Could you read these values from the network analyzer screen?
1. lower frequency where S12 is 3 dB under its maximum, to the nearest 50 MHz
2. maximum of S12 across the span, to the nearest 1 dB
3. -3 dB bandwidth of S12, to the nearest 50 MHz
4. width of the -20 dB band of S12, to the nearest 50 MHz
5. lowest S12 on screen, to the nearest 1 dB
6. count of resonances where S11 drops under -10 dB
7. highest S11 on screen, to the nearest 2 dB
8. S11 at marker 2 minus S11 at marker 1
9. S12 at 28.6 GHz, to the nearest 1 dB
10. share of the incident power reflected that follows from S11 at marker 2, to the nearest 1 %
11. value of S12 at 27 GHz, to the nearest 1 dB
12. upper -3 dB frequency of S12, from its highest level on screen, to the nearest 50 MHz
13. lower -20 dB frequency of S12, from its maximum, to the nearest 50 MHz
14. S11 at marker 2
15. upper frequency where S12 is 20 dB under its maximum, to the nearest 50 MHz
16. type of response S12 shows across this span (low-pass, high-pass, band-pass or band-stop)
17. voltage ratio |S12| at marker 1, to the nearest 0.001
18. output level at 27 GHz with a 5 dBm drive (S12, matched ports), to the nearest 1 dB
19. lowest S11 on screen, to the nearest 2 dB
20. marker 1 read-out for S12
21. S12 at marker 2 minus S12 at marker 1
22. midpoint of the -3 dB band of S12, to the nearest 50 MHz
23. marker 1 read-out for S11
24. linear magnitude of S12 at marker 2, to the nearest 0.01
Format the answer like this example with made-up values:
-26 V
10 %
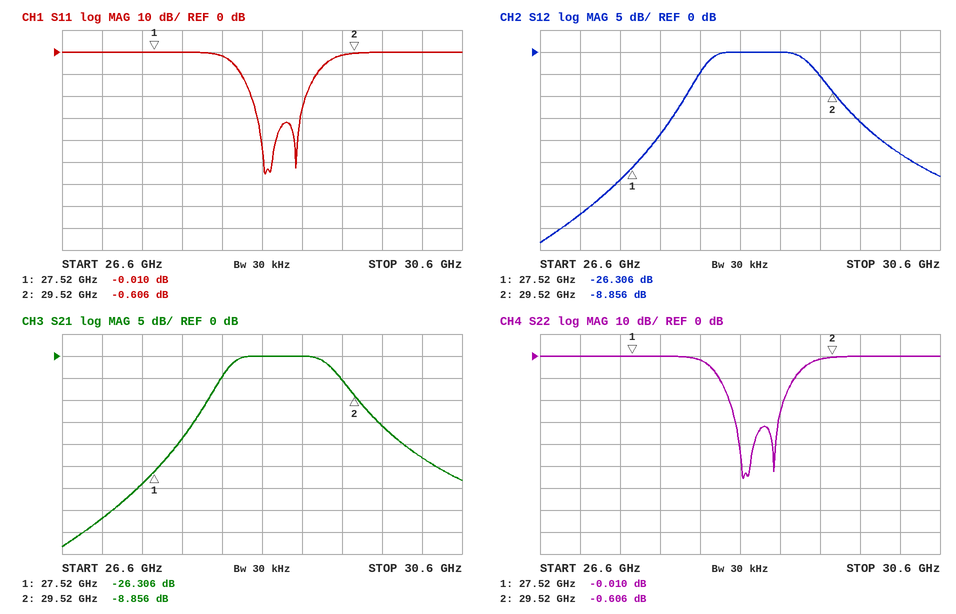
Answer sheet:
28.25 GHz
0 dB
1.05 GHz
2.25 GHz
-43 dB
2
0 dB
-0.596 dB
0 dB
87 %
-37 dB
29.30 GHz
27.75 GHz
-0.606 dB
30.00 GHz
band-pass
0.048
-32 dBm
-56 dB
-26.306 dB
17.450 dB
28.80 GHz
-0.010 dB
0.36
